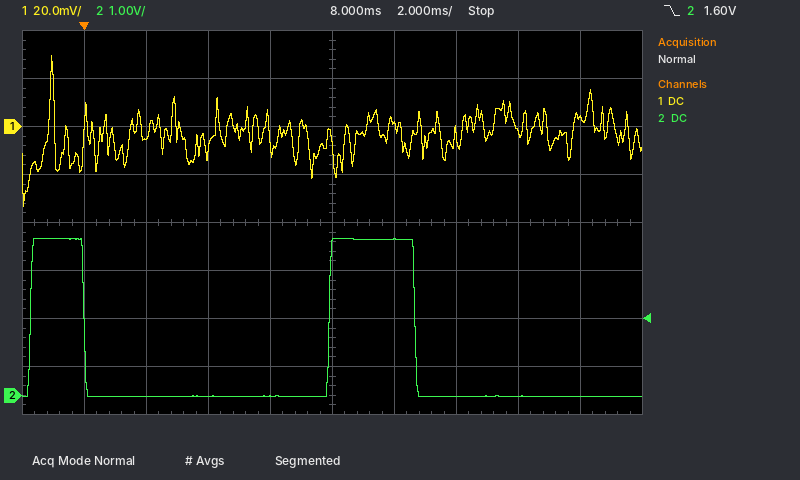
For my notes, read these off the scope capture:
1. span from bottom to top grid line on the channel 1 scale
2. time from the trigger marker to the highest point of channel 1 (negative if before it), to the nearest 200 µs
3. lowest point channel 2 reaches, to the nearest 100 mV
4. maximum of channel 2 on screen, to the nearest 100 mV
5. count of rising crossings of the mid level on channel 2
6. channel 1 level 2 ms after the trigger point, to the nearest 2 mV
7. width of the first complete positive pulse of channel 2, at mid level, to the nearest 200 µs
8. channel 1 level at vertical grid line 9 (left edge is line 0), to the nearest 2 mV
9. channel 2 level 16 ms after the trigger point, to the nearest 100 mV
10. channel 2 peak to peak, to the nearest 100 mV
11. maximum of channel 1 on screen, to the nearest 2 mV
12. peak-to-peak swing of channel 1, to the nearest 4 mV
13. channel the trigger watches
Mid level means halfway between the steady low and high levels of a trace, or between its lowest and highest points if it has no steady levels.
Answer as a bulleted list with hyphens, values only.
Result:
- 160 mV
- -1.0 ms
- 0.0 V
- 3.3 V
- 2
- -4 mV
- 1.8 ms
- 4 mV
- 0.0 V
- 3.3 V
- 30 mV
- 64 mV
- channel 2
